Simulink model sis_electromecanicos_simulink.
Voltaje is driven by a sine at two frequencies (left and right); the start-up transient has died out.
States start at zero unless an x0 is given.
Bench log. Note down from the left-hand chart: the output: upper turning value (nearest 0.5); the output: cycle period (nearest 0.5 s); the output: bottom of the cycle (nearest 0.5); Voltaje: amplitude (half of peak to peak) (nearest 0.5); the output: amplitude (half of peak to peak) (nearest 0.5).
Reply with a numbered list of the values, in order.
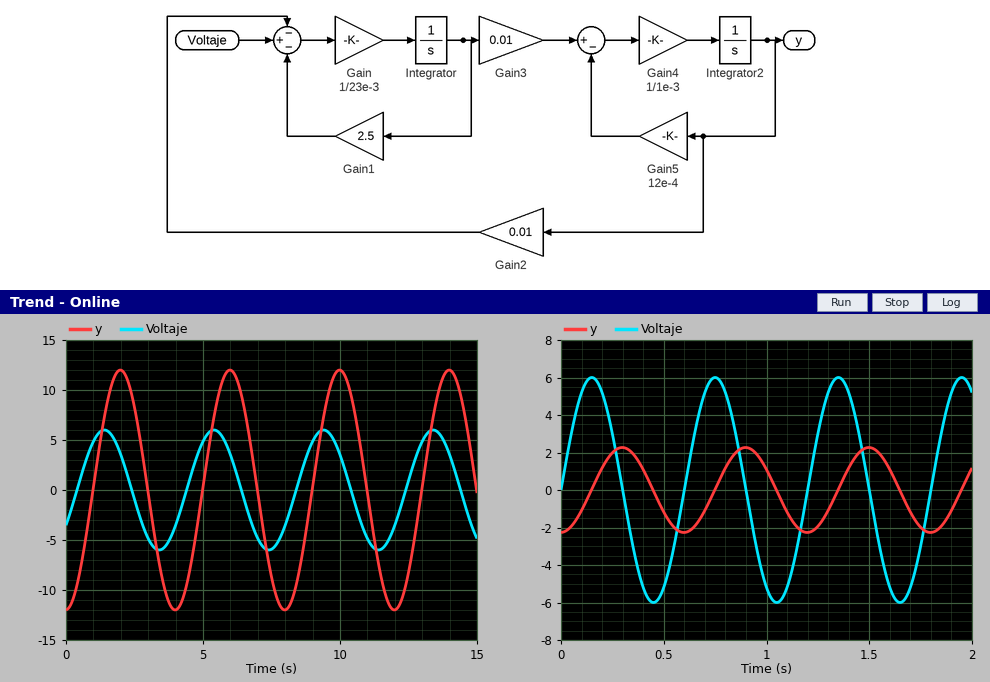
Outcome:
1. 12.0
2. 4.0 s
3. -12.0
4. 6.0
5. 12.0
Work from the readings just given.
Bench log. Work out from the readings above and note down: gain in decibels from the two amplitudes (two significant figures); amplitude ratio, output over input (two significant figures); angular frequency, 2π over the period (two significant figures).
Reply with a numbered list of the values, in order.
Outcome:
1. 6.0 dB
2. 2.0
3. 1.6 rad/s
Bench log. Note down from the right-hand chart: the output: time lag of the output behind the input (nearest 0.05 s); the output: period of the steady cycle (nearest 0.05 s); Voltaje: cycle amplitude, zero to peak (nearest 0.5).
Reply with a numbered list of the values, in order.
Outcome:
1. 0.15 s
2. 0.60 s
3. 6.0
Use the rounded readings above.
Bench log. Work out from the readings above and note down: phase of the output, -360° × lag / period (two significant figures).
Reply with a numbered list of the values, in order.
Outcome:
1. -90°
